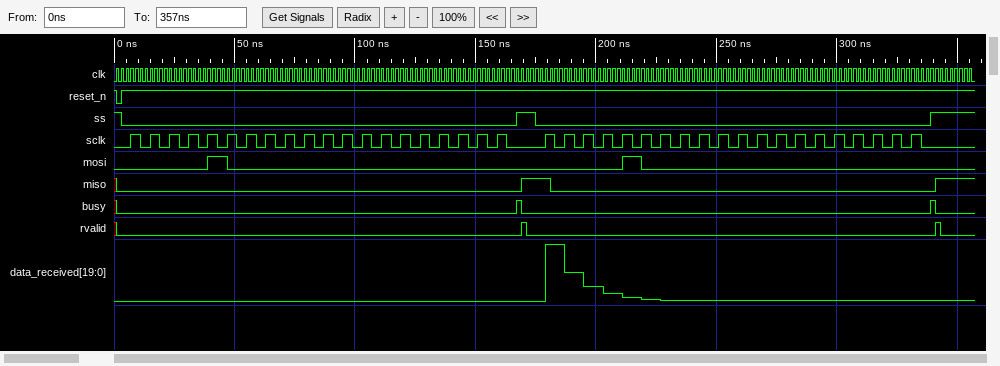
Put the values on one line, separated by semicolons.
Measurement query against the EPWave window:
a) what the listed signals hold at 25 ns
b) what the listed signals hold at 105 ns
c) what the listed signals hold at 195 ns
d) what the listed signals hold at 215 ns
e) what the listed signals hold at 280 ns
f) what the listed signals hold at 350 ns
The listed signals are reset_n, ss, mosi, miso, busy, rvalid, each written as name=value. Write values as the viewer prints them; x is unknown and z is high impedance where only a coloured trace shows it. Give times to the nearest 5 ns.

reset_n=1, ss=0, mosi=0, miso=0, busy=0, rvalid=0; reset_n=1, ss=0, mosi=0, miso=0, busy=0, rvalid=0; reset_n=1, ss=0, mosi=0, miso=0, busy=0, rvalid=0; reset_n=1, ss=0, mosi=1, miso=0, busy=0, rvalid=0; reset_n=1, ss=0, mosi=0, miso=0, busy=0, rvalid=0; reset_n=1, ss=1, mosi=0, miso=1, busy=0, rvalid=0
